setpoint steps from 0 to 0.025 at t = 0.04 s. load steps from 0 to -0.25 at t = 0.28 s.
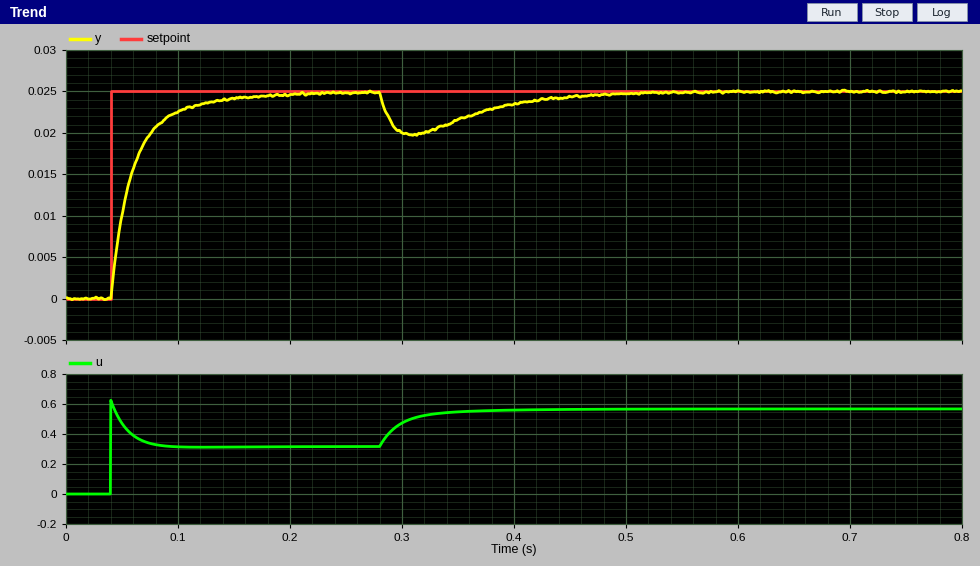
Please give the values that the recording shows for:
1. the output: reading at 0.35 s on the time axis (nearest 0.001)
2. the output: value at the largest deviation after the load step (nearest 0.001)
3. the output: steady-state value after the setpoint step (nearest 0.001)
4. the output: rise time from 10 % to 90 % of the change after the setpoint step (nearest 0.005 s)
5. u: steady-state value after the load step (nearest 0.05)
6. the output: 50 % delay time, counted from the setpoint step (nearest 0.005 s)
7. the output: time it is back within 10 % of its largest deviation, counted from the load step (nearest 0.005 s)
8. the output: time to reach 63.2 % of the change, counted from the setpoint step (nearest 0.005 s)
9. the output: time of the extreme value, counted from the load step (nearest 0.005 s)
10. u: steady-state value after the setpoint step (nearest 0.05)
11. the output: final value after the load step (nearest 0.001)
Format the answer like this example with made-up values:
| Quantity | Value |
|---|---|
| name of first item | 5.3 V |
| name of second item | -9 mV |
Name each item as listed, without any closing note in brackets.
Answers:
| Quantity | Value |
|---|---|
| the output: reading at 0.35 s on the time axis | 0.022 |
| the output: value at the largest deviation after the load step | 0.020 |
| the output: steady-state value after the setpoint step | 0.025 |
| the output: rise time from 10 % to 90 % of the change after the setpoint step | 0.055 s |
| u: steady-state value after the load step | 0.55 |
| the output: 50 % delay time, counted from the setpoint step | 0.015 s |
| the output: time it is back within 10 % of its largest deviation, counted from the load step | 0.185 s |
| the output: time to reach 63.2 % of the change, counted from the setpoint step | 0.020 s |
| the output: time of the extreme value, counted from the load step | 0.030 s |
| u: steady-state value after the setpoint step | 0.30 |
| the output: final value after the load step | 0.025 |
